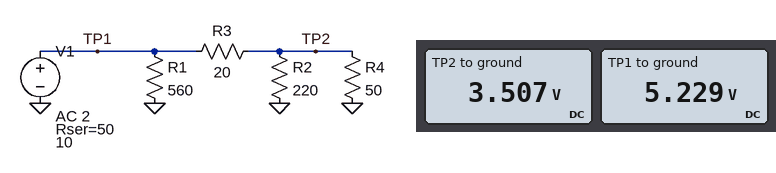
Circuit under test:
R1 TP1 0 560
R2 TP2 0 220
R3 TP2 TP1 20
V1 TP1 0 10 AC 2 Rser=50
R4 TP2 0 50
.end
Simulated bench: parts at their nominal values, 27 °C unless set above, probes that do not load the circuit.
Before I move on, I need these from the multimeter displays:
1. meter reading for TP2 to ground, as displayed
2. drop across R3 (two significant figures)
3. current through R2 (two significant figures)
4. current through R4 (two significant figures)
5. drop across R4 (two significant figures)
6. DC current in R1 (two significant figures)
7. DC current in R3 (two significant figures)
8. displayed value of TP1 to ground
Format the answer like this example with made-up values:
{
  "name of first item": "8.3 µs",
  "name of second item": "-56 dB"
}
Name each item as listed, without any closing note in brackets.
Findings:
{
  "meter reading for TP2 to ground, as displayed": "3.507 V",
  "drop across R3": "1.7 V",
  "current through R2": "16 mA",
  "current through R4": "70 mA",
  "drop across R4": "3.5 V",
  "DC current in R1": "9.3 mA",
  "DC current in R3": "86 mA",
  "displayed value of TP1 to ground": "5.229 V"
}
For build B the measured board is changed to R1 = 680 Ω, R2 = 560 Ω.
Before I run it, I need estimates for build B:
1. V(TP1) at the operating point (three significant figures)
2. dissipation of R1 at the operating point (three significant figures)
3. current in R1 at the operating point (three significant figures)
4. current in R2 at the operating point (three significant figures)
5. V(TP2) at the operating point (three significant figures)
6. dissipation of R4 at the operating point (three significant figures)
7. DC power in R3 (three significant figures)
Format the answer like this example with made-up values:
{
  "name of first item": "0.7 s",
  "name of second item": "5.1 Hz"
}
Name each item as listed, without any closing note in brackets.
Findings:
{
  "V(TP1) at the operating point": "5.46 V",
  "dissipation of R1 at the operating point": "43.8 mW",
  "current in R1 at the operating point": "8.03 mA",
  "current in R2 at the operating point": "6.79 mA",
  "V(TP2) at the operating point": "3.80 V",
  "dissipation of R4 at the operating point": "289 mW",
  "DC power in R3": "137 mW"
}
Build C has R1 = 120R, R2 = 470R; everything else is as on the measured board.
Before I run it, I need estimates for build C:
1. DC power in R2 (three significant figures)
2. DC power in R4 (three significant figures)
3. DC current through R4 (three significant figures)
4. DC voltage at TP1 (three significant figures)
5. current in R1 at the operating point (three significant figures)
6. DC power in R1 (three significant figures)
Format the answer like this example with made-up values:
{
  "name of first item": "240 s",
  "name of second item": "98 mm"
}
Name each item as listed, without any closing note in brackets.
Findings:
{
  "DC power in R2": "21.4 mW",
  "DC power in R4": "202 mW",
  "DC current through R4": "63.5 mA",
  "DC voltage at TP1": "4.58 V",
  "current in R1 at the operating point": "38.2 mA",
  "DC power in R1": "175 mW"
}
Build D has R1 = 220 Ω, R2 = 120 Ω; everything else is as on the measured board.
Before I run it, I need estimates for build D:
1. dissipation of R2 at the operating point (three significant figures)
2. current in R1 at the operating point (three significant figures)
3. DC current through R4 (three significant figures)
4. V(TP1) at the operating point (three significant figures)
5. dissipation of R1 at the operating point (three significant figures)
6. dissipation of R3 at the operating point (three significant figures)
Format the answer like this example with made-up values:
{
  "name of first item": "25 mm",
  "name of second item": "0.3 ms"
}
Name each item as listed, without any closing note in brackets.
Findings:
{
  "dissipation of R2 at the operating point": "74.7 mW",
  "current in R1 at the operating point": "21.3 mA",
  "DC current through R4": "59.9 mA",
  "V(TP1) at the operating point": "4.69 V",
  "dissipation of R1 at the operating point": "100 mW",
  "dissipation of R3 at the operating point": "144 mW"
}
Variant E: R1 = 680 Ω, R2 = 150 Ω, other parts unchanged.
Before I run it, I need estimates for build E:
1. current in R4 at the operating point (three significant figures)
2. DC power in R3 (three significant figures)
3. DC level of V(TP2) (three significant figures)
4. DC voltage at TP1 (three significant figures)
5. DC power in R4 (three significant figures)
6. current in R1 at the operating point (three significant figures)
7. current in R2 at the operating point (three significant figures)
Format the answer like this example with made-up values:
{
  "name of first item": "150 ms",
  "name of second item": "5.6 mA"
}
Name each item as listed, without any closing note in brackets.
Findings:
{
  "current in R4 at the operating point": "67.1 mA",
  "DC power in R3": "160 mW",
  "DC level of V(TP2)": "3.36 V",
  "DC voltage at TP1": "5.15 V",
  "DC power in R4": "225 mW",
  "current in R1 at the operating point": "7.57 mA",
  "current in R2 at the operating point": "22.4 mA"
}
